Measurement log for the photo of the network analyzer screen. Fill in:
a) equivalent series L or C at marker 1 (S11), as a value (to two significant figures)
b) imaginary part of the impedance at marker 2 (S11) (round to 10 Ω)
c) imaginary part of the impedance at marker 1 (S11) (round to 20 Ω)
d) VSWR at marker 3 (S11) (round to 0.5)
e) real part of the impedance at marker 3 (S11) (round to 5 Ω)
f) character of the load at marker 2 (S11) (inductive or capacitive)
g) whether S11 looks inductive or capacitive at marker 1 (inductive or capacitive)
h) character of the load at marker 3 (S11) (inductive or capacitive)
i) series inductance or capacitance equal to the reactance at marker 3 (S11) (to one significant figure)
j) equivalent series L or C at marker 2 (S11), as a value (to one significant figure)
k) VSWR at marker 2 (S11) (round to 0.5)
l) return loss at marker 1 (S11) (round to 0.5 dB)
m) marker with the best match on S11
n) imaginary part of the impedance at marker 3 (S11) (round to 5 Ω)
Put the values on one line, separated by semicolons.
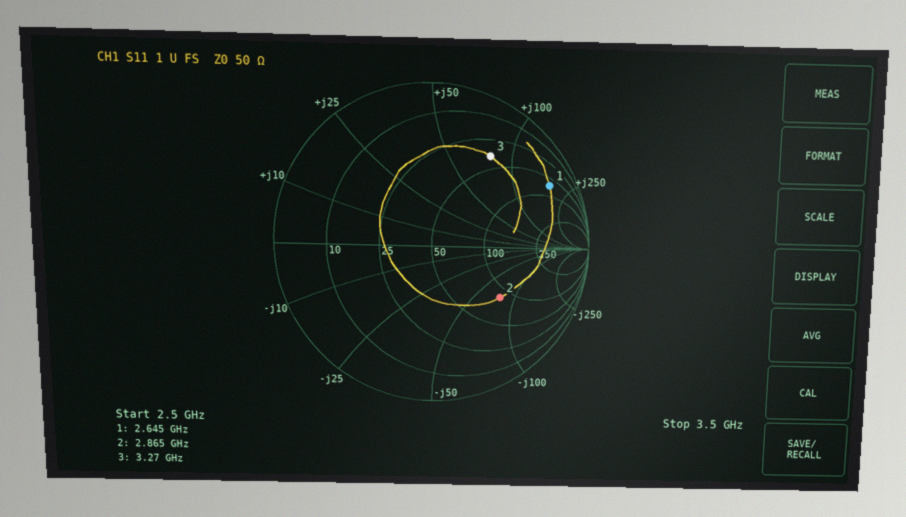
11 nH; -80 Ω; +180 Ω; 5.0; 40 Ω; capacitive; inductive; inductive; 4 nH; 700 fF; 3.5; 1.5 dB; marker 2; +80 Ω
